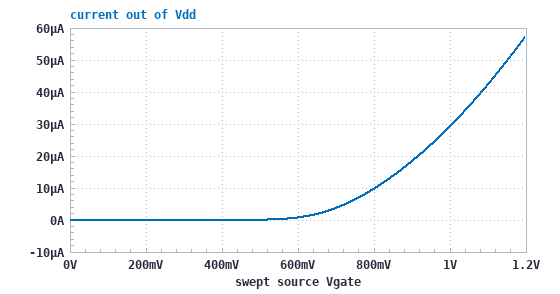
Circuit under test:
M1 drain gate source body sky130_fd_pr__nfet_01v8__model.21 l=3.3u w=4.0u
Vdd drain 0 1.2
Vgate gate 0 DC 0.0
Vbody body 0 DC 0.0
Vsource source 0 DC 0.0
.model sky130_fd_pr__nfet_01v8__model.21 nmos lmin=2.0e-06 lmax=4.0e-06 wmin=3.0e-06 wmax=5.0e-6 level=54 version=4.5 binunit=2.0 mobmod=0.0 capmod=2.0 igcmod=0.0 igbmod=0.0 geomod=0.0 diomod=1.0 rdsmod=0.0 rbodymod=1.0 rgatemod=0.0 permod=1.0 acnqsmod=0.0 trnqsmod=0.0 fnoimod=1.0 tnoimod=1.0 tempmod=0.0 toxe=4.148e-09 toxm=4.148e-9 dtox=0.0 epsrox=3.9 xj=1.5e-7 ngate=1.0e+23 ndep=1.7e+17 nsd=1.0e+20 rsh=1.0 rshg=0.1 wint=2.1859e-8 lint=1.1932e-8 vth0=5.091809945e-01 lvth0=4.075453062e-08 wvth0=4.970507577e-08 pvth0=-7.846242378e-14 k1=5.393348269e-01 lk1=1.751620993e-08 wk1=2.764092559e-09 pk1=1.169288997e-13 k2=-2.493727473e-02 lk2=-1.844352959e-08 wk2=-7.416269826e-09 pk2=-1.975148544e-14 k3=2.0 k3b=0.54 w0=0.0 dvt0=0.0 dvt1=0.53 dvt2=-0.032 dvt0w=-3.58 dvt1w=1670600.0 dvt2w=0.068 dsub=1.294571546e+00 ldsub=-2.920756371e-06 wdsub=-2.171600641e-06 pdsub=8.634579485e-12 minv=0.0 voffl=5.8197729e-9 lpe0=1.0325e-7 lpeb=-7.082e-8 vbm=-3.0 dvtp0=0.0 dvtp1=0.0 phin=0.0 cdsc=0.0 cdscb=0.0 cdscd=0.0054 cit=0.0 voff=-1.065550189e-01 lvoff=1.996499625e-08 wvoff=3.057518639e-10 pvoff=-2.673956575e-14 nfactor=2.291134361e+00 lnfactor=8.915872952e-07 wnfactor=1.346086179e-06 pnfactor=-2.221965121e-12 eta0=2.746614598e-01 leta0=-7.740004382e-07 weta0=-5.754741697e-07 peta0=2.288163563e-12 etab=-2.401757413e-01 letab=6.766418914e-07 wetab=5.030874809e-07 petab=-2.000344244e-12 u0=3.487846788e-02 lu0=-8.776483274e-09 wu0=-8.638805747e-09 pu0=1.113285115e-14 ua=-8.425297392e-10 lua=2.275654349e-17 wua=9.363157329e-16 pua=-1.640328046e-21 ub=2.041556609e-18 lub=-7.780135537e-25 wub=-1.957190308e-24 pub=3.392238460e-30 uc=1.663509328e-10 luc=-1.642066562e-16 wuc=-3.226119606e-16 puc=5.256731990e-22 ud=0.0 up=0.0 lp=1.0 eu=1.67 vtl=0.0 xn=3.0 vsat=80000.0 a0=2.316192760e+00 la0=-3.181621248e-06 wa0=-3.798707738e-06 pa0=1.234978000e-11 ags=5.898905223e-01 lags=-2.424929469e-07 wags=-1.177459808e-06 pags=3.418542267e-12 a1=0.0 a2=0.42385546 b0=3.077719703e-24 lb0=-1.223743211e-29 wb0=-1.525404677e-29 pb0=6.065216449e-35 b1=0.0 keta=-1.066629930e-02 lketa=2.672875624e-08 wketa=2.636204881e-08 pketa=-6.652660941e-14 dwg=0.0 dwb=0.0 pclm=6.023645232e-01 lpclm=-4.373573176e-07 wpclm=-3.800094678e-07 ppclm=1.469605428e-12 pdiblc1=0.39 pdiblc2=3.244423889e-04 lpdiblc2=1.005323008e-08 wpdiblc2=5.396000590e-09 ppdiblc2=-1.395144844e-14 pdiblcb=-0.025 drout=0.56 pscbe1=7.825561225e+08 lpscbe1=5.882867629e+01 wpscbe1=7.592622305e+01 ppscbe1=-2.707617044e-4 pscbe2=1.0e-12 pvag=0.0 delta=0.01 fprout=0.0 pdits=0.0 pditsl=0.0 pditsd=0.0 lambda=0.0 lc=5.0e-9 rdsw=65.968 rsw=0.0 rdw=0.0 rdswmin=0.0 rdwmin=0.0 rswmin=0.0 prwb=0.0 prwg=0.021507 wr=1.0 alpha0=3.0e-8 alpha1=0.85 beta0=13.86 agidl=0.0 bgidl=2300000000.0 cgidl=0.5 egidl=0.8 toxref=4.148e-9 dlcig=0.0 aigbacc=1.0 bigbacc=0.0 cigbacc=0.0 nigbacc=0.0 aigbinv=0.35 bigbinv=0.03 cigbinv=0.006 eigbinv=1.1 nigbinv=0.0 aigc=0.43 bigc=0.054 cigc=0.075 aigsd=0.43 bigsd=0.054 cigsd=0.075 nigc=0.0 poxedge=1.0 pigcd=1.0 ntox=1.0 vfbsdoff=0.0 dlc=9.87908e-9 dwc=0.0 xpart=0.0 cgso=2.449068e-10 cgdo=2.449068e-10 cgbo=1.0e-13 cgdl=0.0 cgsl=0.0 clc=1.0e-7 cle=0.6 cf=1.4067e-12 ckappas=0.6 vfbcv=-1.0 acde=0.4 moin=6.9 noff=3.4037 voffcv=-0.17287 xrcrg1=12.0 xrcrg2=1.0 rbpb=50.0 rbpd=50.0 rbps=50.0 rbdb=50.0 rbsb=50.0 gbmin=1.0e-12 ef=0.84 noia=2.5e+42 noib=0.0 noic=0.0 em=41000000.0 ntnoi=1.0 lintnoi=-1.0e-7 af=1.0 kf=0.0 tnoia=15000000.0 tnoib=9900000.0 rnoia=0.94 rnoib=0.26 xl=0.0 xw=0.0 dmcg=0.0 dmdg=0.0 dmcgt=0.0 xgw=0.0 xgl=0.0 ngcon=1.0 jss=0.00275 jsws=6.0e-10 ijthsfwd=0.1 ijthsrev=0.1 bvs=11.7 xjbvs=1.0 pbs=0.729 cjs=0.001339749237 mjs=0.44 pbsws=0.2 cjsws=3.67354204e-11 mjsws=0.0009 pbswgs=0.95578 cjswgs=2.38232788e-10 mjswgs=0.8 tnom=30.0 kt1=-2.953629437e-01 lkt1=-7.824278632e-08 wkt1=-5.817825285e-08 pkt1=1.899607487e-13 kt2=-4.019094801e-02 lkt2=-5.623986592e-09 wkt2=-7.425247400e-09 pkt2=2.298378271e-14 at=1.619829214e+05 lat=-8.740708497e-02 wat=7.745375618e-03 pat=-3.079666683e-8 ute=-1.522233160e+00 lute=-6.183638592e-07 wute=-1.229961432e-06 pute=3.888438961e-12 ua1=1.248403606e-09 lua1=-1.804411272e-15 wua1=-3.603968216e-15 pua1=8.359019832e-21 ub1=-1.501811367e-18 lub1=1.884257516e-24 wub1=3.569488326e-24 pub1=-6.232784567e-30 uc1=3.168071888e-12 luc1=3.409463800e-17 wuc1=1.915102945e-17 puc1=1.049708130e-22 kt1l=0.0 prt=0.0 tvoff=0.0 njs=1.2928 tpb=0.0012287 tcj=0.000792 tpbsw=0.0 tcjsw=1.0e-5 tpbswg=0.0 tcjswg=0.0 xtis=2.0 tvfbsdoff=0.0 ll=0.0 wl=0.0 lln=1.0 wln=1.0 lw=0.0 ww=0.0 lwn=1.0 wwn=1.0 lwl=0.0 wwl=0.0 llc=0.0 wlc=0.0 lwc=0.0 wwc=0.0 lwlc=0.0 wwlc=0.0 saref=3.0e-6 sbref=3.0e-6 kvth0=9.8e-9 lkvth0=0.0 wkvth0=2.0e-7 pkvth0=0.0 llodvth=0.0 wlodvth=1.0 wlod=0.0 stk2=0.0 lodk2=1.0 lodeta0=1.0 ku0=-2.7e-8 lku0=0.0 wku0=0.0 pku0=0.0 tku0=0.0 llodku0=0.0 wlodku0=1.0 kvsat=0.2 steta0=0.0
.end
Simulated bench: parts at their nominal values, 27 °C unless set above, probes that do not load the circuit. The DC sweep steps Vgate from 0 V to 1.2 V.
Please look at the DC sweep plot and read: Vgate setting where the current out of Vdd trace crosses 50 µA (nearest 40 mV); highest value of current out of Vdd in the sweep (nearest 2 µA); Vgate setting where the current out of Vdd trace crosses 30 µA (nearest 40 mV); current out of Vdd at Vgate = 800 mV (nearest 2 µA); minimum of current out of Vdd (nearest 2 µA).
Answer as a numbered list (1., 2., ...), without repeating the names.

1. 1.16 V
2. 58 µA
3. 1.00 V
4. 10 µA
5. 0 A
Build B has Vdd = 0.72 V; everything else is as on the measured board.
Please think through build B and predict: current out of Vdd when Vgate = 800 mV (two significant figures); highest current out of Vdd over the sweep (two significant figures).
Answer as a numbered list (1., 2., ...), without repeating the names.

1. 9.7 µA
2. 57 µA
